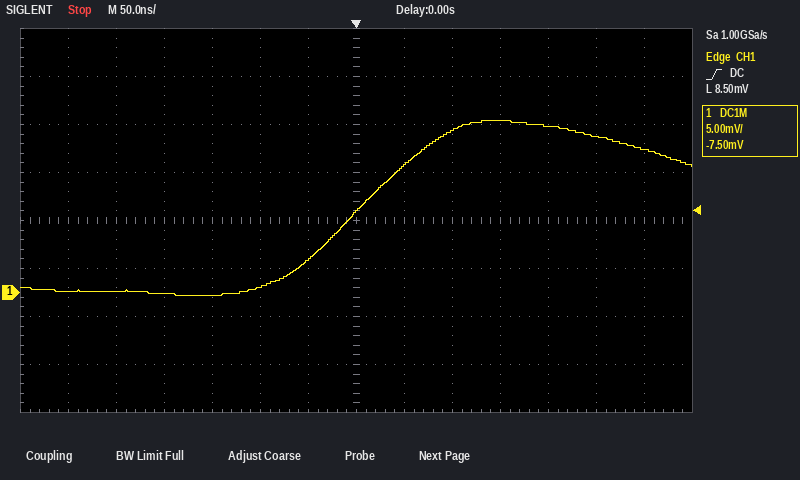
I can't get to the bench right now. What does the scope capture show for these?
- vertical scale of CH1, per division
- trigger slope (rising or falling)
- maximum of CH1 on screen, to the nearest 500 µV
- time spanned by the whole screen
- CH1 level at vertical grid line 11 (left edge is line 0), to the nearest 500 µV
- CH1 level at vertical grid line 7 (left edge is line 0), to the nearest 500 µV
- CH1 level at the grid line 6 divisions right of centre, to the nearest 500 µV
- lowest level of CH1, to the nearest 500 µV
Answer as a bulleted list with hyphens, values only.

- 5 mV
- rising
- 18.0 mV
- 700 ns
- 17.5 mV
- 8.5 mV
- 15.0 mV
- -500 µV
